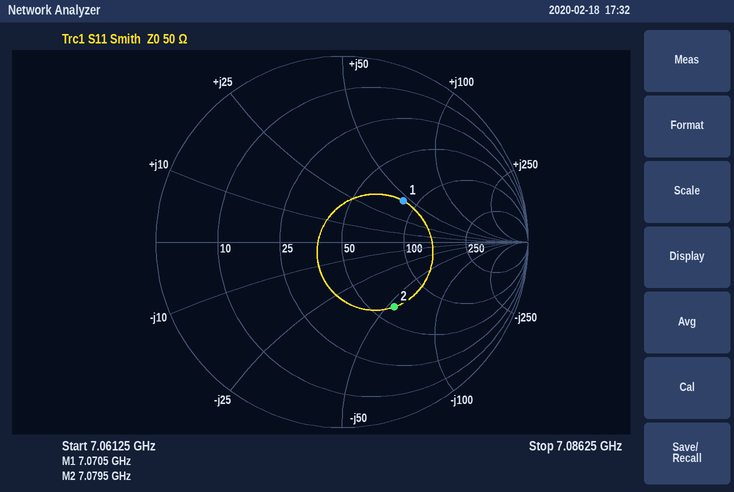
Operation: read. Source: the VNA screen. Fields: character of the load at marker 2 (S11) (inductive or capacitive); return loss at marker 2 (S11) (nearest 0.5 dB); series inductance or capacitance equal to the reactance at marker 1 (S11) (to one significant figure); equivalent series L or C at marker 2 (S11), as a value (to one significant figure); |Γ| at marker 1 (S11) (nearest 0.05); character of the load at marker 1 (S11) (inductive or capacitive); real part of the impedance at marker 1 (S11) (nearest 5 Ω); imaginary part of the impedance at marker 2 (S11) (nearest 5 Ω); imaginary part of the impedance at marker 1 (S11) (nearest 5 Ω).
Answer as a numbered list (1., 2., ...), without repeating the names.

1. capacitive
2. 7.0 dB
3. 1.0 nH
4. 400 fF
5. 0.40
6. inductive
7. 85 Ω
8. -55 Ω
9. +45 Ω
